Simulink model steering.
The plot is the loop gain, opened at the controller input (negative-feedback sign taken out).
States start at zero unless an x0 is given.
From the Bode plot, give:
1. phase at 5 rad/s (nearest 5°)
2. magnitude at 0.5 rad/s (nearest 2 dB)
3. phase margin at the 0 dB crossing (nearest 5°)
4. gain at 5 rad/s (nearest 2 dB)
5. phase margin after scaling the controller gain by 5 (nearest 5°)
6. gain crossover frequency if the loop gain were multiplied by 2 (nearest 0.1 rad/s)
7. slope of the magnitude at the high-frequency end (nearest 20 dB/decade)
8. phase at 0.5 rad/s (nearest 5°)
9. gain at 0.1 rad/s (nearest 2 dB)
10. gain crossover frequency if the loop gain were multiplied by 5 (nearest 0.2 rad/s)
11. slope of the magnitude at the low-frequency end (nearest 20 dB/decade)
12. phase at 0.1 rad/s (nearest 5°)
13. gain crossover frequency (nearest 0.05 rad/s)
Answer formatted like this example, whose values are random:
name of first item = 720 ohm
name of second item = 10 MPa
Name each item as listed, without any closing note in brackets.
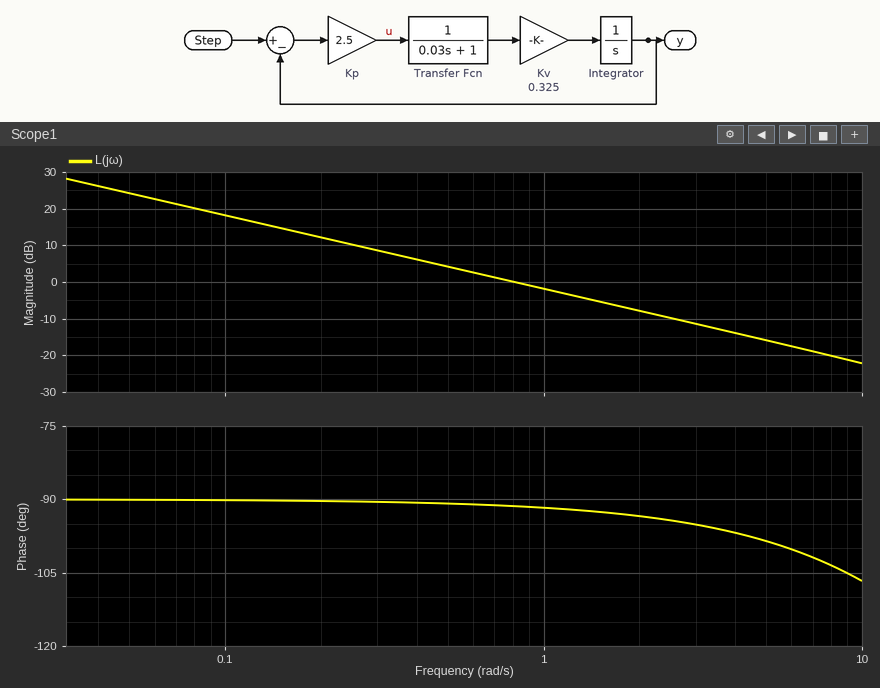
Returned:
phase at 5 rad/s = -100°
magnitude at 0.5 rad/s = 4 dB
phase margin at the 0 dB crossing = 90°
gain at 5 rad/s = -16 dB
phase margin after scaling the controller gain by 5 = 85°
gain crossover frequency if the loop gain were multiplied by 2 = 1.6 rad/s
slope of the magnitude at the high-frequency end = -20 dB/decade
phase at 0.5 rad/s = -90°
gain at 0.1 rad/s = 18 dB
gain crossover frequency if the loop gain were multiplied by 5 = 4.0 rad/s
slope of the magnitude at the low-frequency end = -20 dB/decade
phase at 0.1 rad/s = -90°
gain crossover frequency = 0.80 rad/s
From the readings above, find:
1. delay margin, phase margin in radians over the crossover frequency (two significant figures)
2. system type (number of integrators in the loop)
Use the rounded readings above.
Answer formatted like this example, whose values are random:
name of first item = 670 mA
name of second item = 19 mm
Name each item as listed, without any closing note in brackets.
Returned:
delay margin, phase margin in radians over the crossover frequency = 2.0 s
system type = 1
